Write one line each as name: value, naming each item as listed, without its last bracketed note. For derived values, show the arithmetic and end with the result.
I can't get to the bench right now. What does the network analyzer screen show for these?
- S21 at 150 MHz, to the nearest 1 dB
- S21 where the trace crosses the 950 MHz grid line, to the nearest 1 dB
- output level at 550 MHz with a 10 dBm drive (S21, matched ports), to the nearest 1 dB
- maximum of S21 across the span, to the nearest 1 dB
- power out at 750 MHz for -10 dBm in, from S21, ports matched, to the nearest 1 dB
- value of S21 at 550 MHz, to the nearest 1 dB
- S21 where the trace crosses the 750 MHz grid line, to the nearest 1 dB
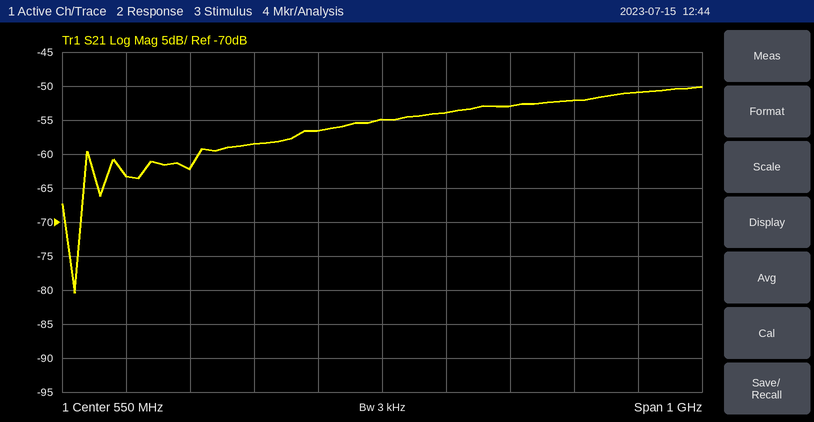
S21 at 150 MHz, to the nearest 1 dB: -63 dB
S21 where the trace crosses the 950 MHz grid line, to the nearest 1 dB: -51 dB
output level at 550 MHz with a 10 dBm drive (S21, matched ports), to the nearest 1 dB: 10 dBm + (-55 dB) = -45 dBm
maximum of S21 across the span, to the nearest 1 dB: -50 dB
power out at 750 MHz for -10 dBm in, from S21, ports matched, to the nearest 1 dB: -10 dBm + (-53 dB) = -63 dBm
value of S21 at 550 MHz, to the nearest 1 dB: -55 dB
S21 where the trace crosses the 750 MHz grid line, to the nearest 1 dB: -53 dB
